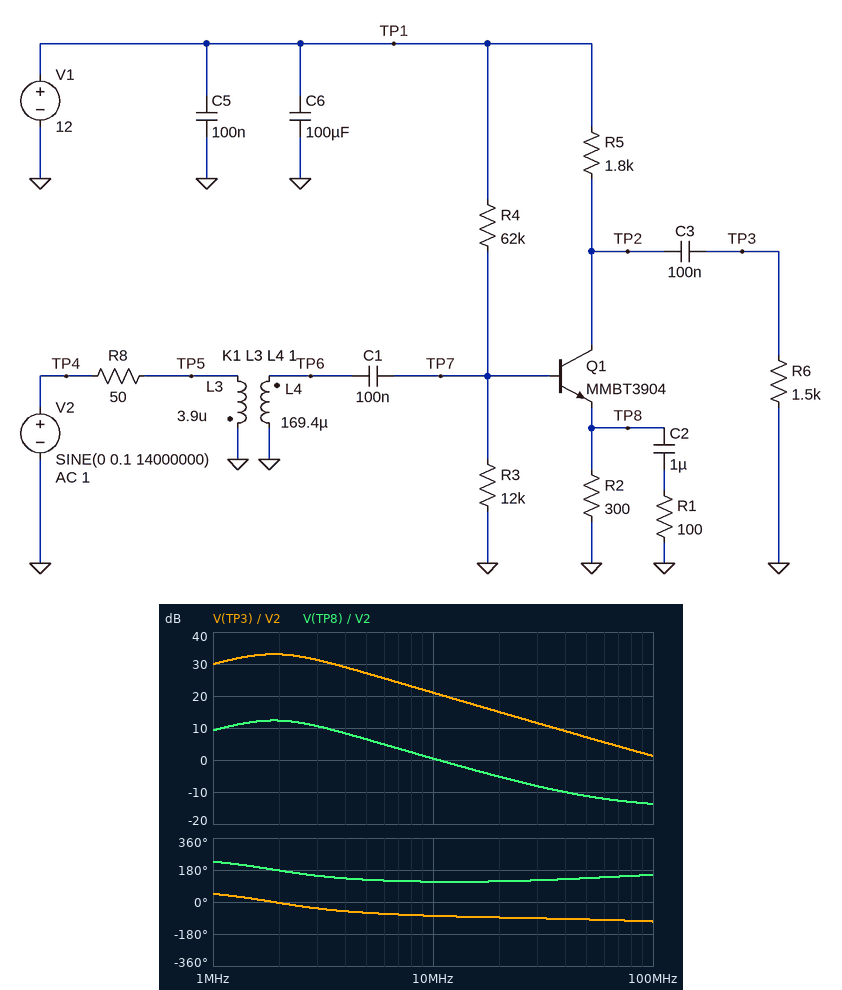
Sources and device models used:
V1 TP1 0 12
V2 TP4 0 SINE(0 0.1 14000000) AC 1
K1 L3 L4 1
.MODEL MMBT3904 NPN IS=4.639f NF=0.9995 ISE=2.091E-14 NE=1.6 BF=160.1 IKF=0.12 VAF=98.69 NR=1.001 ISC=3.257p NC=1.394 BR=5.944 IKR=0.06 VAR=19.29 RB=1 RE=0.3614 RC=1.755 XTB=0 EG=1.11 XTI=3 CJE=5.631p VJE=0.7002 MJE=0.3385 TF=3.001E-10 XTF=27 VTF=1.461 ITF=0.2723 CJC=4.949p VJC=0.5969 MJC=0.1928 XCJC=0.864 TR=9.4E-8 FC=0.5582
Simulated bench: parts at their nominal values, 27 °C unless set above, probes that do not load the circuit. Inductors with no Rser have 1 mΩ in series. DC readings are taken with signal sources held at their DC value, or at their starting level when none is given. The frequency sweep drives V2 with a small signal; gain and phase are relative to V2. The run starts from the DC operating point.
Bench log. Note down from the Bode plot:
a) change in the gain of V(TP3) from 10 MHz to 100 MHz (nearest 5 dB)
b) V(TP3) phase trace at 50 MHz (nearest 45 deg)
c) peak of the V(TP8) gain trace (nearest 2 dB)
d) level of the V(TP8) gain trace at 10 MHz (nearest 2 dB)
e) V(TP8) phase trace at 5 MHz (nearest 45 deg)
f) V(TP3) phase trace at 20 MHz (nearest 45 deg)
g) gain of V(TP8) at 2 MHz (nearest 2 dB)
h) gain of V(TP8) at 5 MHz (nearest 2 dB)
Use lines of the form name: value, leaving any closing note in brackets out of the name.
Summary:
change in the gain of V(TP3) from 10 MHz to 100 MHz: -20 dB
V(TP3) phase trace at 50 MHz: -90 deg
peak of the V(TP8) gain trace: 12 dB
level of the V(TP8) gain trace at 10 MHz: 0 dB
V(TP8) phase trace at 5 MHz: 135 deg
V(TP3) phase trace at 20 MHz: -90 deg
gain of V(TP8) at 2 MHz: 12 dB
gain of V(TP8) at 5 MHz: 6 dB
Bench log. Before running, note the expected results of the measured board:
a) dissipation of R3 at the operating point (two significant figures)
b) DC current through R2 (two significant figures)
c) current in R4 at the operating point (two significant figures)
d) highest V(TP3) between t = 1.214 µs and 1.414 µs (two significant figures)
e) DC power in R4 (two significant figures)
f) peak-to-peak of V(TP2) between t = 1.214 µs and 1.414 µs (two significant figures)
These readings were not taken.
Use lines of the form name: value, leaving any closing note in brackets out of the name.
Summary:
dissipation of R3 at the operating point: 250 µW
DC current through R2: 3.4 mA
current in R4 at the operating point: 170 µA
highest V(TP3) between t = 1.214 µs and 1.414 µs: 800 mV
DC power in R4: 1.7 mW
peak-to-peak of V(TP2) between t = 1.214 µs and 1.414 µs: 1.6 V
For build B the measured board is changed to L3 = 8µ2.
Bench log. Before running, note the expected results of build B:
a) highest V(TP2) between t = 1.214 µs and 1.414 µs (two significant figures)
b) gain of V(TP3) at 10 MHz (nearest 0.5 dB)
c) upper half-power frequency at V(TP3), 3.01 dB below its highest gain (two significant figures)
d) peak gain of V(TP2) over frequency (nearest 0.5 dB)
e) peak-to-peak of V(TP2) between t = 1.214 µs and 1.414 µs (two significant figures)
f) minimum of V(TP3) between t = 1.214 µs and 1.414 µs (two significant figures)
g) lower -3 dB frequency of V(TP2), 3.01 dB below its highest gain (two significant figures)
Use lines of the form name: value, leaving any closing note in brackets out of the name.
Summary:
highest V(TP2) between t = 1.214 µs and 1.414 µs: 7.0 V
gain of V(TP3) at 10 MHz: 23.5 dB
upper half-power frequency at V(TP3), 3.01 dB below its highest gain: 5.0 MHz
peak gain of V(TP2) over frequency: 31.5 dB
peak-to-peak of V(TP2) between t = 1.214 µs and 1.414 µs: 2.2 V
minimum of V(TP3) between t = 1.214 µs and 1.414 µs: -1.1 V
lower -3 dB frequency of V(TP2), 3.01 dB below its highest gain: 690 kHz
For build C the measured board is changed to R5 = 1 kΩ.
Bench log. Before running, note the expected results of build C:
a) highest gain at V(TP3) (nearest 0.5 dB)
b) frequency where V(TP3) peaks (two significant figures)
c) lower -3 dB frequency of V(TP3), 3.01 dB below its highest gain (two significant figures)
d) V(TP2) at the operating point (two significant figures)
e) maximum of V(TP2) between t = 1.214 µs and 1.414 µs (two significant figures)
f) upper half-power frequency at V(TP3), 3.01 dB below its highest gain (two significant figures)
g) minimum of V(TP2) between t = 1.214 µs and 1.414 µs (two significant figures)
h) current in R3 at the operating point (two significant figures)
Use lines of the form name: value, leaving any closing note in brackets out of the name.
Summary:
highest gain at V(TP3): 30.5 dB
frequency where V(TP3) peaks: 2.2 MHz
lower -3 dB frequency of V(TP3), 3.01 dB below its highest gain: 1.1 MHz
V(TP2) at the operating point: 8.6 V
maximum of V(TP2) between t = 1.214 µs and 1.414 µs: 9.4 V
upper half-power frequency at V(TP3), 3.01 dB below its highest gain: 4.5 MHz
minimum of V(TP2) between t = 1.214 µs and 1.414 µs: 7.8 V
current in R3 at the operating point: 140 µA
